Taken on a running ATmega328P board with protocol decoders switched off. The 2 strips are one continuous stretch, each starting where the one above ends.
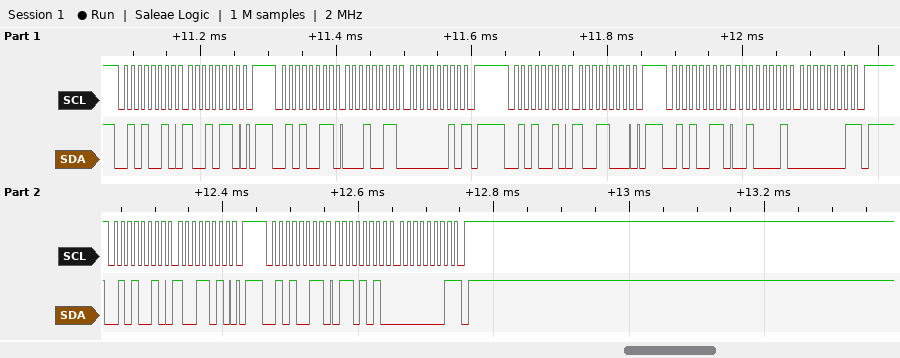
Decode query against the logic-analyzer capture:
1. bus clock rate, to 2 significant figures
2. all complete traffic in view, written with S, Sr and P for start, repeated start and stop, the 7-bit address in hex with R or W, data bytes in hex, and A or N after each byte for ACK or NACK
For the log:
100 kHz
S 29W A 96 A P S 29R A 13 A 02 N P S 29W A 98 A P S 29R A 21 A 01 N P S 29W A 9A A P S 29R A 6A A 01 N P
